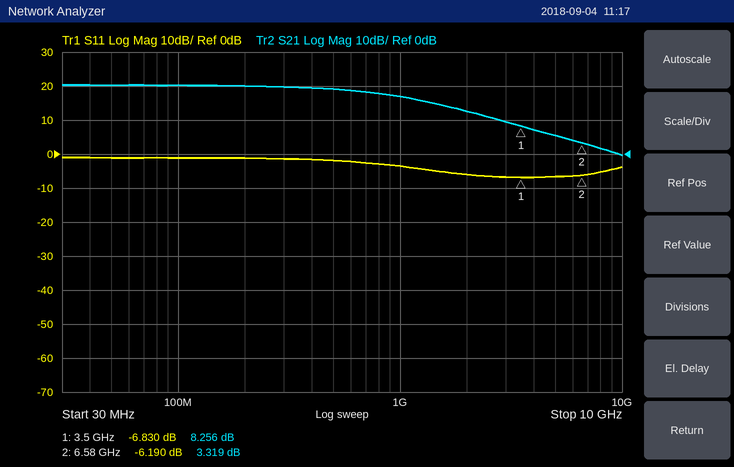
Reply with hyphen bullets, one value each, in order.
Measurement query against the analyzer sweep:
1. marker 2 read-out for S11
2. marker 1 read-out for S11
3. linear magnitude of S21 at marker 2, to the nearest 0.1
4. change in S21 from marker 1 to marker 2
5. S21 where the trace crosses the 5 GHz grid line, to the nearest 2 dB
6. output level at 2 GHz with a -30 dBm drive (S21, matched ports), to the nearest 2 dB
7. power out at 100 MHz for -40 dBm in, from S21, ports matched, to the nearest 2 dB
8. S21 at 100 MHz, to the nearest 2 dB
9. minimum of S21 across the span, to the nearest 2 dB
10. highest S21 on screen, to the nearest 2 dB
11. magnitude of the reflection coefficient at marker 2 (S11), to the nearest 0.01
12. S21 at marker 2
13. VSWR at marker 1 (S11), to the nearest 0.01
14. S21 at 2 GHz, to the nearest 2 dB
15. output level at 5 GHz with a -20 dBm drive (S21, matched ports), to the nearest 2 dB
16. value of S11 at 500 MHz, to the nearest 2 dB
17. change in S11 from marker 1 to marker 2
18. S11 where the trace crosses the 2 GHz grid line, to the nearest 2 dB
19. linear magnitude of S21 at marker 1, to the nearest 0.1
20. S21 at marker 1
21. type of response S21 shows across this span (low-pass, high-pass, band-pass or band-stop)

- -6.190 dB
- -6.830 dB
- 1.5
- -4.937 dB
- 6 dB
- -18 dBm
- -20 dBm
- 20 dB
- 0 dB
- 20 dB
- 0.49
- 3.319 dB
- 2.67
- 12 dB
- -14 dBm
- -2 dB
- 0.640 dB
- -6 dB
- 2.6
- 8.256 dB
- low-pass
